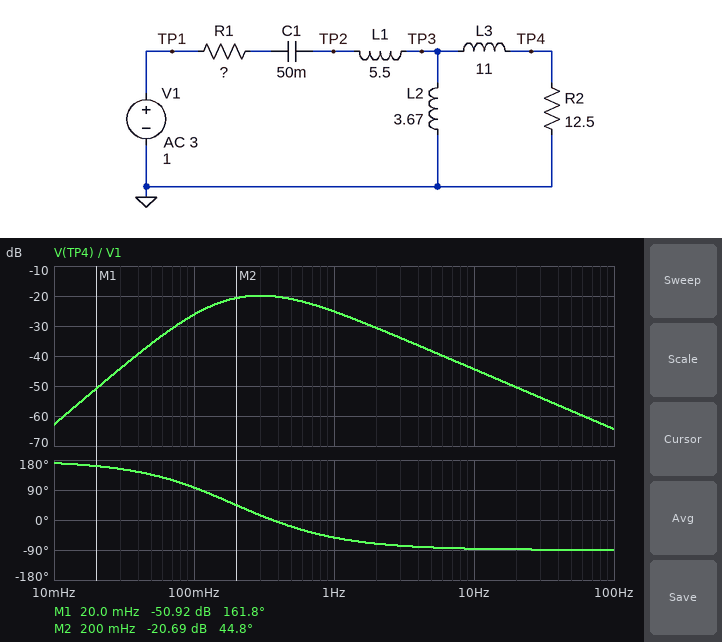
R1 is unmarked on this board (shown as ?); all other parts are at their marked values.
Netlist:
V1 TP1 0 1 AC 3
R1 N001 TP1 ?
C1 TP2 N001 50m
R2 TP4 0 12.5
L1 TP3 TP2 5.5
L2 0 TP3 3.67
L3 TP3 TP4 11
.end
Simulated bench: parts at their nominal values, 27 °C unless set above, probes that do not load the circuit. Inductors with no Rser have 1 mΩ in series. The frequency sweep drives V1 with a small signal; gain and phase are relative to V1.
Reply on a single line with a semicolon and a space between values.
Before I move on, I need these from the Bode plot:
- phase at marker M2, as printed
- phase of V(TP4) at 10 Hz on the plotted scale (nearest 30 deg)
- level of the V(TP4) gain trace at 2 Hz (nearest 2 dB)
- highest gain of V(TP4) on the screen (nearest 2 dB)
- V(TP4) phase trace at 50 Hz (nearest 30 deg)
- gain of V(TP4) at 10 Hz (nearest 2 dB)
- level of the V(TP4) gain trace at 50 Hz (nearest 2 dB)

44.8 deg; -90 deg; -30 dB; -20 dB; -90 deg; -44 dB; -58 dB
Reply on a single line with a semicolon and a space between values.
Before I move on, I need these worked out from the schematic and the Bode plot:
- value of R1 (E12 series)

27 Ω
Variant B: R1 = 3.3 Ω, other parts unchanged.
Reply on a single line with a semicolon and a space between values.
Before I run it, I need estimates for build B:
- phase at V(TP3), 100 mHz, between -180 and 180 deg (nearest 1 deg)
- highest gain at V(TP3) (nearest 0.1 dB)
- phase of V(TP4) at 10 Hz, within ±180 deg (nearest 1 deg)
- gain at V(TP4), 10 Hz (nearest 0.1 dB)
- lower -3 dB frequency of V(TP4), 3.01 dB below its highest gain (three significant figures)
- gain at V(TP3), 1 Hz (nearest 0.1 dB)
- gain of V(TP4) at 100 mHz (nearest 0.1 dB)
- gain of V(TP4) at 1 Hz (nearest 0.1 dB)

165 deg; 1.5 dB; -89 deg; -44.4 dB; 212 mHz; -9.0 dB; -23.1 dB; -24.0 dB
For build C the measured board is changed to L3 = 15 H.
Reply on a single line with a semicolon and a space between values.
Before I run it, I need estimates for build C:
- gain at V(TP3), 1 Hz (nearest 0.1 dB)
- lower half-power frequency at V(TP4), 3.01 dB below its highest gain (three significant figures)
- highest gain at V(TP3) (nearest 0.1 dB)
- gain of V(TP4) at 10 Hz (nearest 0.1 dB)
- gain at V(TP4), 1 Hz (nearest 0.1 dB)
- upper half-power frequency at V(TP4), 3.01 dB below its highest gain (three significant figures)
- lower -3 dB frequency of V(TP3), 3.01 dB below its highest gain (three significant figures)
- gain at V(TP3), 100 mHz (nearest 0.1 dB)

-9.7 dB; 130 mHz; -9.1 dB; -46.7 dB; -27.4 dB; 670 mHz; 399 mHz; -25.1 dB
